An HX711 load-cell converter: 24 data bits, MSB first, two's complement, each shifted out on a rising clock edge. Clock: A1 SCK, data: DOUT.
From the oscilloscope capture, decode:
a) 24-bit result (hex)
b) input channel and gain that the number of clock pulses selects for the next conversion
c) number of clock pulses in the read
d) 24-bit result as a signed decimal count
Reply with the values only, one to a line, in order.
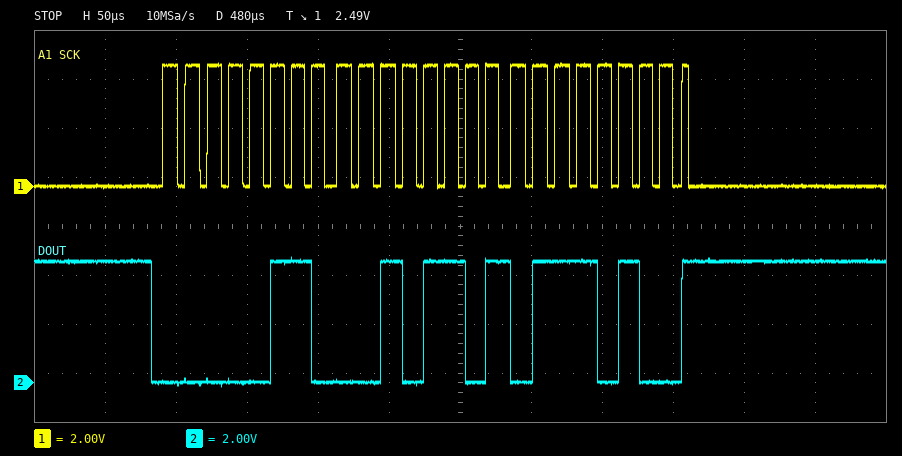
0x062D74
channel A, gain 128
25
404852
